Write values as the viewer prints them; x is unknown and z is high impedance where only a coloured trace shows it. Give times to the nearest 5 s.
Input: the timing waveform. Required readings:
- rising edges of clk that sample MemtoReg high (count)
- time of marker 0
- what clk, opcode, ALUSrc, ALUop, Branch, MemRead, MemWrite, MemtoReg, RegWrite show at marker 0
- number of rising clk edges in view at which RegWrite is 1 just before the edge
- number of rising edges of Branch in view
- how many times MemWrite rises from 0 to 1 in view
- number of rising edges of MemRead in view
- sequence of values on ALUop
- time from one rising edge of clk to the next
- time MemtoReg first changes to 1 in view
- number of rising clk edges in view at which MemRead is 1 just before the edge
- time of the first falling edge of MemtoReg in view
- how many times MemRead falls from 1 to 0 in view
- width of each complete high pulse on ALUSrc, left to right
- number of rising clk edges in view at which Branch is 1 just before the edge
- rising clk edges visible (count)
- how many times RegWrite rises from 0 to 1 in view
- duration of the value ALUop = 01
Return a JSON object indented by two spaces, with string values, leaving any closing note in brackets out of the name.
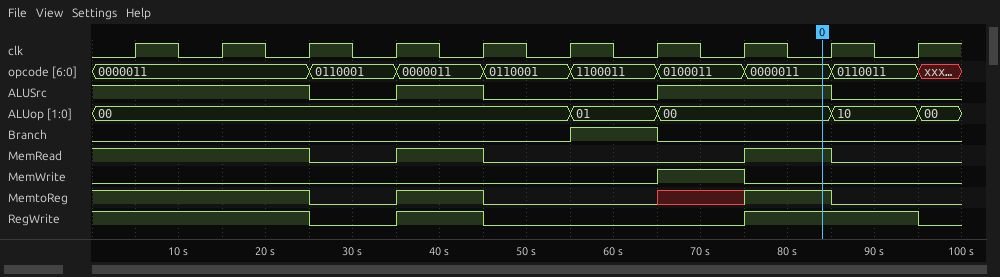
{
  "rising edges of clk that sample MemtoReg high": "5",
  "time of marker 0": "85 s",
  "what clk, opcode, ALUSrc, ALUop, Branch, MemRead, MemWrite, MemtoReg, RegWrite show at marker 0": "clk=0, opcode=0000011, ALUSrc=1, ALUop=00, Branch=0, MemRead=1, MemWrite=0, MemtoReg=1, RegWrite=1",
  "number of rising clk edges in view at which RegWrite is 1 just before the edge": "6",
  "number of rising edges of Branch in view": "1",
  "how many times MemWrite rises from 0 to 1 in view": "1",
  "number of rising edges of MemRead in view": "2",
  "sequence of values on ALUop": "00, 01, 00, 10, 00",
  "time from one rising edge of clk to the next": "10 s",
  "time MemtoReg first changes to 1 in view": "35 s",
  "number of rising clk edges in view at which MemRead is 1 just before the edge": "5",
  "time of the first falling edge of MemtoReg in view": "25 s",
  "how many times MemRead falls from 1 to 0 in view": "3",
  "width of each complete high pulse on ALUSrc, left to right": "10 s, 20 s",
  "number of rising clk edges in view at which Branch is 1 just before the edge": "1",
  "rising clk edges visible": "10",
  "how many times RegWrite rises from 0 to 1 in view": "2",
  "duration of the value ALUop = 01": "10 s"
}
